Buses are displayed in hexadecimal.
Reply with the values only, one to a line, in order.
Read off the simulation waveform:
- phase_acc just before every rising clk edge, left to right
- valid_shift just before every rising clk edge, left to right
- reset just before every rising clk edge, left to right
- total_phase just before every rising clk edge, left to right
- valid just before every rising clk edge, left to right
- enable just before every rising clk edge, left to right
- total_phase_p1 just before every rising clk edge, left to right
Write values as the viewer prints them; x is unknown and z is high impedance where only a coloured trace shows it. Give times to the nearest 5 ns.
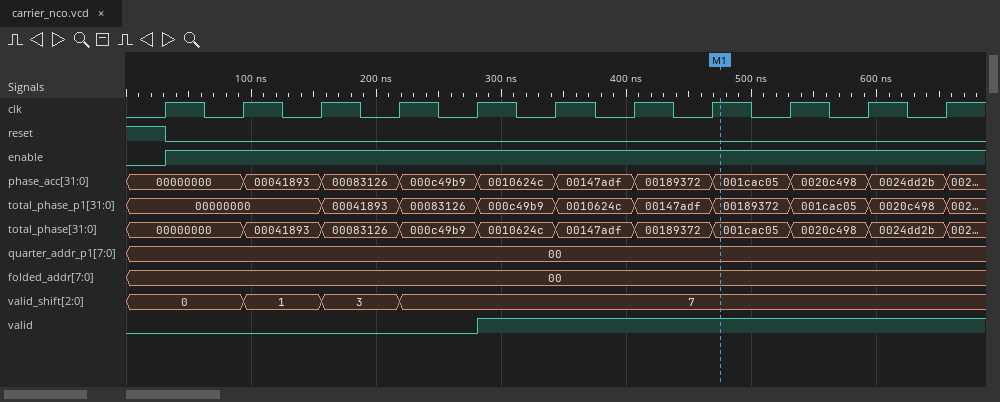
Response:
00000000, 00000000, 00041893, 00083126, 000c49b9, 0010624c, 00147adf, 00189372, 001cac05, 0020c498, 0024dd2b
0, 0, 1, 3, 7, 7, 7, 7, 7, 7, 7
1 0 0 0 0 0 0 0 0 0 0
00000000, 00000000, 00041893, 00083126, 000c49b9, 0010624c, 00147adf, 00189372, 001cac05, 0020c498, 0024dd2b
0 0 0 0 0 1 1 1 1 1 1
0 1 1 1 1 1 1 1 1 1 1
00000000, 00000000, 00000000, 00041893, 00083126, 000c49b9, 0010624c, 00147adf, 00189372, 001cac05, 0020c498
